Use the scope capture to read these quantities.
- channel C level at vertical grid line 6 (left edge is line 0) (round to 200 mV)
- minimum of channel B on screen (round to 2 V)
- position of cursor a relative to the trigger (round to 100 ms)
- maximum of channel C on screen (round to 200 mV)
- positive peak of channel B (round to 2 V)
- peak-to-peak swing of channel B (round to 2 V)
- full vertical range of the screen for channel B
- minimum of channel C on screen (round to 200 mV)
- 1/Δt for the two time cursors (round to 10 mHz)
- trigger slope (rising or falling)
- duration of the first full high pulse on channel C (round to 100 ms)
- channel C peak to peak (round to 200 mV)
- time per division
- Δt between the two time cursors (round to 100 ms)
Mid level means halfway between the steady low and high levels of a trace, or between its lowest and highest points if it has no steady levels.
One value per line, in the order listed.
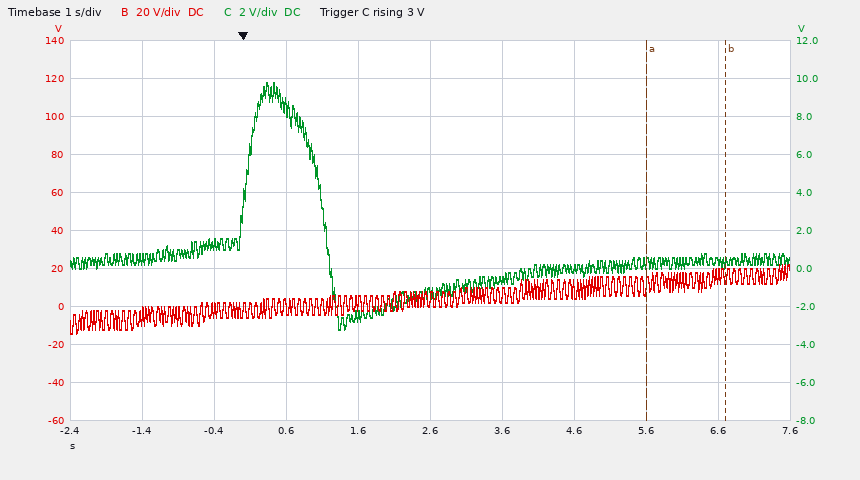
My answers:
-600 mV
-14 V
+5.6 s
9.8 V
22 V
36 V
200 V
-3.2 V
910 mHz
rising
1.1 s
13.0 V
1 s
1.1 s
